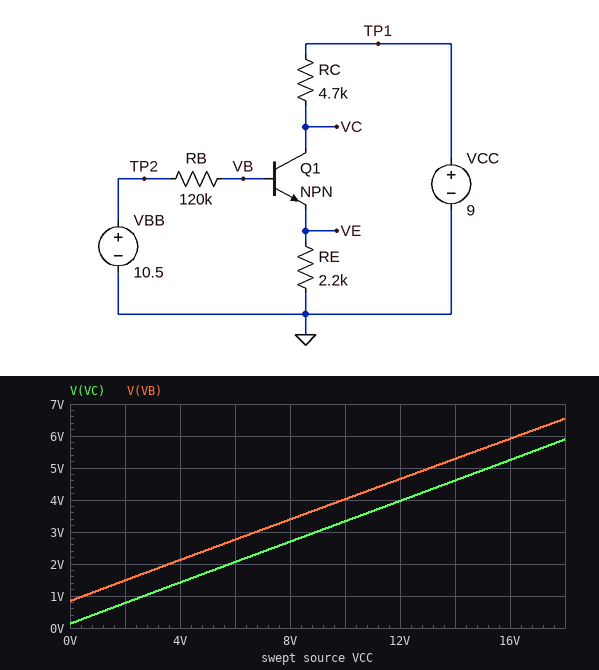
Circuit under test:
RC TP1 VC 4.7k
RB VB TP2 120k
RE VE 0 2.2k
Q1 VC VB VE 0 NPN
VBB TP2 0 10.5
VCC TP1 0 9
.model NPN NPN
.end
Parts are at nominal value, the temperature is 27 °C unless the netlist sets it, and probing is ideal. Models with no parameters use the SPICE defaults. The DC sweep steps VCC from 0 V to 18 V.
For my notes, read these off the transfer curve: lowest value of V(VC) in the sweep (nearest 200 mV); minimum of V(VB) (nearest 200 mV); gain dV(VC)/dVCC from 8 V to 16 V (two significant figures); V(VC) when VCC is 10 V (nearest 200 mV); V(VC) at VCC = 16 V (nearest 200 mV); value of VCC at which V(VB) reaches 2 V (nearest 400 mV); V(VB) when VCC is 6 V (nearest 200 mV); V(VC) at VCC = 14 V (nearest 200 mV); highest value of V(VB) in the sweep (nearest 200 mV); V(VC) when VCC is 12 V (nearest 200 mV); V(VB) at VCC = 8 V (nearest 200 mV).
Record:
200 mV
800 mV
0.32 V/V
3.4 V
5.2 V
3.6 V
2.8 V
4.6 V
6.6 V
4.0 V
3.4 V
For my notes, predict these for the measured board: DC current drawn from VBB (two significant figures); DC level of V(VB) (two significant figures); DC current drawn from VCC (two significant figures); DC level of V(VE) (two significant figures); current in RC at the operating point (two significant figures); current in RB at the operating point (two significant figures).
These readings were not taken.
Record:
57 µA
3.7 V
1.3 mA
2.9 V
1.3 mA
57 µA
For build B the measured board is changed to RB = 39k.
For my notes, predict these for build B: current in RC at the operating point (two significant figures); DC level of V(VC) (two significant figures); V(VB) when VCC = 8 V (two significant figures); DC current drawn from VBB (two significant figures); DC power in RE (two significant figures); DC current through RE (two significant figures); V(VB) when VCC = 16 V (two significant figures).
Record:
1.2 mA
3.2 V
3.6 V
170 µA
4.4 mW
1.4 mA
6.0 V
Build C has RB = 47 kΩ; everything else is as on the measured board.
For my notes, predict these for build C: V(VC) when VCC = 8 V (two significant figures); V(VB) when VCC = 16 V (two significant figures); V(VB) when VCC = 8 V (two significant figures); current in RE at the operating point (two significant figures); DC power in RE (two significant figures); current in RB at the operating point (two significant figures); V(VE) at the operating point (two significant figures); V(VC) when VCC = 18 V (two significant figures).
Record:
2.8 V
6.0 V
3.5 V
1.4 mA
4.3 mW
140 µA
3.1 V
5.9 V
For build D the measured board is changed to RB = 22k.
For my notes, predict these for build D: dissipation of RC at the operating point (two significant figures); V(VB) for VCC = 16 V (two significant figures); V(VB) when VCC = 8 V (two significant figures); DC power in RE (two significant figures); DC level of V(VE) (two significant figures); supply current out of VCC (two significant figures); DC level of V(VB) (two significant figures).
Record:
6.8 mW
6.2 V
3.8 V
4.9 mW
3.3 V
1.2 mA
4.1 V
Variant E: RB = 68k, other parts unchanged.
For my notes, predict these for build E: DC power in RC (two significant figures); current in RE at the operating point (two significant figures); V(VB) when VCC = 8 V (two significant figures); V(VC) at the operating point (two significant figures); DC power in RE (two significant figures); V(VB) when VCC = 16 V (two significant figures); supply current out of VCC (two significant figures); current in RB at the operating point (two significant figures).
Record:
7.5 mW
1.4 mA
3.5 V
3.1 V
4.1 mW
6.0 V
1.3 mA
99 µA
